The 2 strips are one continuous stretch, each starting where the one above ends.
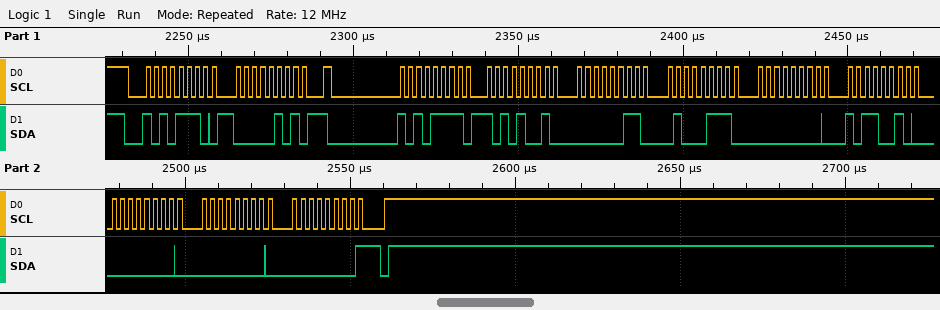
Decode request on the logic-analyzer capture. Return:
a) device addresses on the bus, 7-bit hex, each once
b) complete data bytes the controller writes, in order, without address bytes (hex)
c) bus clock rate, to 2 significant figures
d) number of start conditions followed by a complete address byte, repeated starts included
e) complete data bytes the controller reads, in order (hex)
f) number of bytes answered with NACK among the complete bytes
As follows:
0x57
05
400 kHz
2
A9 03 47 00 B2 00 00 00
1
